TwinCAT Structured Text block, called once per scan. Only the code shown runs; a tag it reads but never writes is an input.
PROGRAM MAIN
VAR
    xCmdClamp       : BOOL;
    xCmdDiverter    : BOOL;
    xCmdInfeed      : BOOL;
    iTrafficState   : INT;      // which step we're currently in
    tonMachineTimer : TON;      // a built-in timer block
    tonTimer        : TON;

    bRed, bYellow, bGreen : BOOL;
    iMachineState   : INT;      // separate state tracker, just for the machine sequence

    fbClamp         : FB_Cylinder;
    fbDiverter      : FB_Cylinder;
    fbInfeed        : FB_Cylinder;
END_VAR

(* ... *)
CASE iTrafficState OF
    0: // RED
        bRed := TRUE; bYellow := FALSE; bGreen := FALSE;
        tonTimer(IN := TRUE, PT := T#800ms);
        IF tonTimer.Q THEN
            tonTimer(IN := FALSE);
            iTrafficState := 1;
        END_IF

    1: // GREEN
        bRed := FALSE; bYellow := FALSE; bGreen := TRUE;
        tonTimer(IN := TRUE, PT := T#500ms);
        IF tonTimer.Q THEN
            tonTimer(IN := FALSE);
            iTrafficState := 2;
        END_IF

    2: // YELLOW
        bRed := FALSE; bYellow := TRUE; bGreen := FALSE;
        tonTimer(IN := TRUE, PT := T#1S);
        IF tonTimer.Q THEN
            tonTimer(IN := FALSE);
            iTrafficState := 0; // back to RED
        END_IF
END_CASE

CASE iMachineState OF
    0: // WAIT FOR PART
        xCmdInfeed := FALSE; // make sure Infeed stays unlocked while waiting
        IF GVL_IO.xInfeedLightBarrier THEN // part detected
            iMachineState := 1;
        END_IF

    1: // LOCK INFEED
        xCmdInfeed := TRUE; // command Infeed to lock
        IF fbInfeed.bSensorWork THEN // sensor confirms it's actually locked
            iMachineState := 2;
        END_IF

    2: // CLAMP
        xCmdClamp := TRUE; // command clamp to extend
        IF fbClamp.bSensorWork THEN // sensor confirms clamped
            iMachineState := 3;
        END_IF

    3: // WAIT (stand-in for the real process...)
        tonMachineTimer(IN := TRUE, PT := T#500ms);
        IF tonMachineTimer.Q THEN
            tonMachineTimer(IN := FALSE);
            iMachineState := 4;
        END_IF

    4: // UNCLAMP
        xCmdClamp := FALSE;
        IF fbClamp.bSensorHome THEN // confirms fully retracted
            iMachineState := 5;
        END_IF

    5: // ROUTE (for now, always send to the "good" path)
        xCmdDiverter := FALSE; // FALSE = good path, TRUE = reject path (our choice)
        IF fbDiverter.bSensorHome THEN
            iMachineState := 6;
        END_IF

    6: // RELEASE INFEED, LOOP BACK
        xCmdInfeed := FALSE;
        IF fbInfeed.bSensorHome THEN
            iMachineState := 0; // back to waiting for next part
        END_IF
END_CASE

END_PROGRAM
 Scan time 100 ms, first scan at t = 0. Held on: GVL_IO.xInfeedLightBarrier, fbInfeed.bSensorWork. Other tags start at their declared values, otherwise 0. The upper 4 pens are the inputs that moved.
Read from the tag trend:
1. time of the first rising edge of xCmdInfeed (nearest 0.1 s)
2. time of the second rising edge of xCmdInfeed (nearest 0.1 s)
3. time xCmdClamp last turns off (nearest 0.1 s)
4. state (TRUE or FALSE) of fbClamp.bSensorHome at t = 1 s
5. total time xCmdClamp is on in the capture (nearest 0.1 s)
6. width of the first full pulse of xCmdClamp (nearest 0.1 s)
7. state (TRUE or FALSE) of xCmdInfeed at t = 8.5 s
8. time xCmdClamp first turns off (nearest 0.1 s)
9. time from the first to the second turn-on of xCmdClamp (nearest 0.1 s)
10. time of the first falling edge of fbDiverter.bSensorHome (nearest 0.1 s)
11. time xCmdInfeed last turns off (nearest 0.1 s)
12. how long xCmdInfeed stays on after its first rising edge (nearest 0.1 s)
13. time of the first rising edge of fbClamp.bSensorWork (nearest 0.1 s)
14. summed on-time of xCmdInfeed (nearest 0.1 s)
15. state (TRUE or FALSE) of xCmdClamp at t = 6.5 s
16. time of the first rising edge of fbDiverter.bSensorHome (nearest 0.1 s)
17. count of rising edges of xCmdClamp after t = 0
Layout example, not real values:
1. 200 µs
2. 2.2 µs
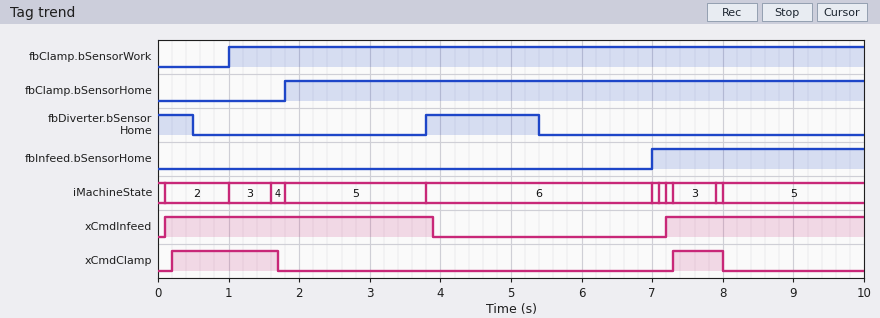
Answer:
1. 0.1 s
2. 7.2 s
3. 8.0 s
4. FALSE
5. 2.2 s
6. 1.5 s
7. TRUE
8. 1.7 s
9. 7.1 s
10. 0.5 s
11. 3.9 s
12. 3.8 s
13. 1.0 s
14. 6.6 s
15. FALSE
16. 3.8 s
17. 2
